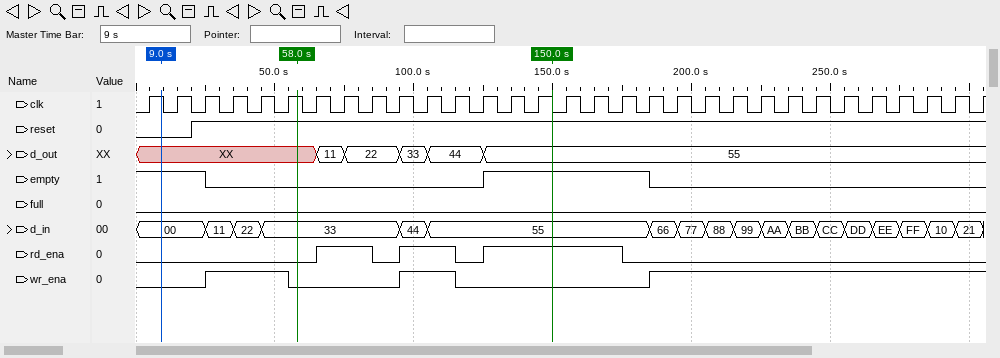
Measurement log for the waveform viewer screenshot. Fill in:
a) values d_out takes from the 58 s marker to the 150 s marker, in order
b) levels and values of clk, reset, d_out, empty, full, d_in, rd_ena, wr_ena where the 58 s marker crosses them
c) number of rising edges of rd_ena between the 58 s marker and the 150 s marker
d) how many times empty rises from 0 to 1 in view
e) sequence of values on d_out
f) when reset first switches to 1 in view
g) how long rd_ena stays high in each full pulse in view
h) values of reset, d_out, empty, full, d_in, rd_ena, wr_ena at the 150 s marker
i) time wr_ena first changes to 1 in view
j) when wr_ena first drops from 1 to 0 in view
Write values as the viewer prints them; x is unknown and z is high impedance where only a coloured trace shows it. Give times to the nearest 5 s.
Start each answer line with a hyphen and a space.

- XX, 11, 22, 33, 44, 55
- clk=1, reset=1, d_out=XX, empty=0, full=0, d_in=33, rd_ena=0, wr_ena=0
- 3
- 1
- XX, 11, 22, 33, 44, 55
- 20 s
- 20 s, 20 s, 50 s
- reset=1, d_out=55, empty=1, full=0, d_in=55, rd_ena=1, wr_ena=0
- 25 s
- 55 s
